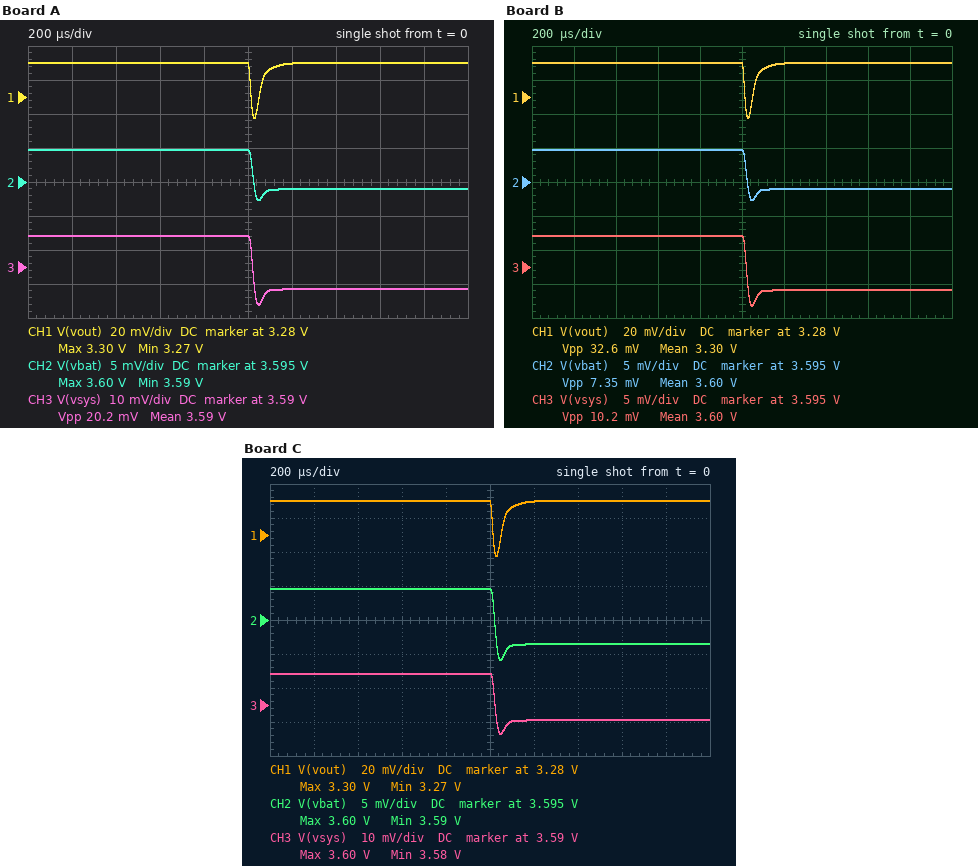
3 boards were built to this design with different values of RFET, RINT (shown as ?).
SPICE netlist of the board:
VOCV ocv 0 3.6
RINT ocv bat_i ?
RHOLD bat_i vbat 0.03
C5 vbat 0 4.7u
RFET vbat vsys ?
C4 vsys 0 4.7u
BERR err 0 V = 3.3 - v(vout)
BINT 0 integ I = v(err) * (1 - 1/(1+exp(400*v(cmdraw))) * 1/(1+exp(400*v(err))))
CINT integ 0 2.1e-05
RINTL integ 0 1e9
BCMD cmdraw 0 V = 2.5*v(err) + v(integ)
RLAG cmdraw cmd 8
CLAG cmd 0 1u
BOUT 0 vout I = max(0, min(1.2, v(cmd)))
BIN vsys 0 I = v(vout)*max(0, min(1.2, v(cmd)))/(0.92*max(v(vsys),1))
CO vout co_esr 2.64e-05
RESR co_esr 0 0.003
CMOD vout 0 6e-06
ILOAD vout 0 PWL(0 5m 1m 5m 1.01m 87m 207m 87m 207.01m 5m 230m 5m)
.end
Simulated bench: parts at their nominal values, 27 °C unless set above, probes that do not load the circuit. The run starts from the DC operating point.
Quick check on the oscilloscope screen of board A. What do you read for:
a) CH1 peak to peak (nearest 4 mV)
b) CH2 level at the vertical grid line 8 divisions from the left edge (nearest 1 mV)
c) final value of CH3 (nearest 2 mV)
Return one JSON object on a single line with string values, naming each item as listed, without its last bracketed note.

{"CH1 peak to peak": "32 mV", "CH2 level at the vertical grid line 8 divisions from the left edge": "3.594 V", "final value of CH3": "3.584 V"}
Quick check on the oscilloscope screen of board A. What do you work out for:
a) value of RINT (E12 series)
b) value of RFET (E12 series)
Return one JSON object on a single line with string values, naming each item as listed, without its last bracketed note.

{"value of RINT": "0.039 Ω", "value of RFET": "0.12 Ω"}
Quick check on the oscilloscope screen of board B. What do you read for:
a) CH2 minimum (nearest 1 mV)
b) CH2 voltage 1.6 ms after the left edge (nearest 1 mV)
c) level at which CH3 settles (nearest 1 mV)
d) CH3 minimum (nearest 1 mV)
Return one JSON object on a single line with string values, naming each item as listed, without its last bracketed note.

{"CH2 minimum": "3.592 V", "CH2 voltage 1.6 ms after the left edge": "3.594 V", "level at which CH3 settles": "3.592 V", "CH3 minimum": "3.589 V"}
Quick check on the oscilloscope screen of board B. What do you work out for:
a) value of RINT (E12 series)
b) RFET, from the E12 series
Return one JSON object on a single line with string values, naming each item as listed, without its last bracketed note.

{"value of RINT": "0.039 Ω", "RFET, from the E12 series": "0.027 Ω"}
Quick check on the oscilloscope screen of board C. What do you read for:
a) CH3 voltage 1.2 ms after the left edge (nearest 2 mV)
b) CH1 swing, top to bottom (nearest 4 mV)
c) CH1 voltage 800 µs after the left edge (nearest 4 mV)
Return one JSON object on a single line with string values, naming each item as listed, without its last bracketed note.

{"CH3 voltage 1.2 ms after the left edge": "3.586 V", "CH1 swing, top to bottom": "32 mV", "CH1 voltage 800 µs after the left edge": "3.300 V"}
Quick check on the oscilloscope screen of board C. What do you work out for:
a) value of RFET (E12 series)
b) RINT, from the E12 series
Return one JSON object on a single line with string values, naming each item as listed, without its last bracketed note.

{"value of RFET": "0.068 Ω", "RINT, from the E12 series": "0.068 Ω"}
